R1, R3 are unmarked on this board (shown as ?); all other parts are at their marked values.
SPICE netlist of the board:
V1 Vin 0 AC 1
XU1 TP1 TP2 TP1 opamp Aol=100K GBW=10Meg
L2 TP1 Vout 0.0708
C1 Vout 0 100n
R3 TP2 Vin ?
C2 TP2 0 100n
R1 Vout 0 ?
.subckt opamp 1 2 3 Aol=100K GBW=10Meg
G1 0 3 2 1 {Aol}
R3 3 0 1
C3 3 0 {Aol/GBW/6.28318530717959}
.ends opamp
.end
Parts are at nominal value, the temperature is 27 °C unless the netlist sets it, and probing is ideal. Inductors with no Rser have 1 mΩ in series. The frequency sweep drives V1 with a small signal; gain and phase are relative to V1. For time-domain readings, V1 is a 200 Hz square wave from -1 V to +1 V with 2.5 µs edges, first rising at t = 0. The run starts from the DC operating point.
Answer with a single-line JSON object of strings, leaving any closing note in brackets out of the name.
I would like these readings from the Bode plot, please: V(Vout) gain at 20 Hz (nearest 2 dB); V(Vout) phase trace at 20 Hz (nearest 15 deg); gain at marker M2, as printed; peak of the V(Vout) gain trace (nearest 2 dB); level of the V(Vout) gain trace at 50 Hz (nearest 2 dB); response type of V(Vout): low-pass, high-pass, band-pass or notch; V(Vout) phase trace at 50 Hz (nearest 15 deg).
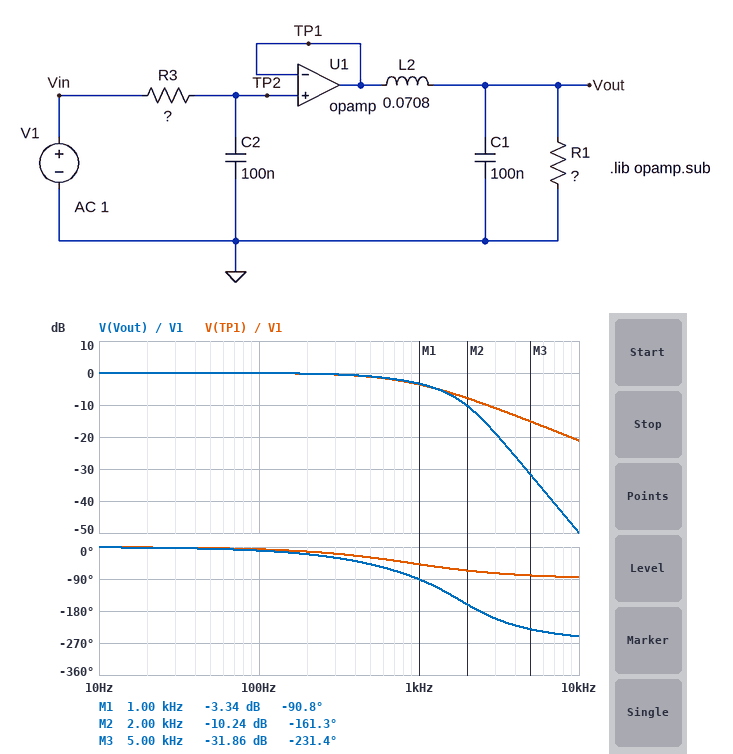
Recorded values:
{"V(Vout) gain at 20 Hz": "0 dB", "V(Vout) phase trace at 20 Hz": "0 deg", "gain at marker M2, as printed": "-10.24 dB", "peak of the V(Vout) gain trace": "0 dB", "level of the V(Vout) gain trace at 50 Hz": "0 dB", "response type of V(Vout): low-pass, high-pass, band-pass or notch": "low-pass", "V(Vout) phase trace at 50 Hz": "0 deg"}
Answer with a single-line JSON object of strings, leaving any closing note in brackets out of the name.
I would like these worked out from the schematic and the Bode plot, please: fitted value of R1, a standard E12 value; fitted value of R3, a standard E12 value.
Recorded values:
{"fitted value of R1, a standard E12 value": "680 Ω", "fitted value of R3, a standard E12 value": "1.8 kΩ"}
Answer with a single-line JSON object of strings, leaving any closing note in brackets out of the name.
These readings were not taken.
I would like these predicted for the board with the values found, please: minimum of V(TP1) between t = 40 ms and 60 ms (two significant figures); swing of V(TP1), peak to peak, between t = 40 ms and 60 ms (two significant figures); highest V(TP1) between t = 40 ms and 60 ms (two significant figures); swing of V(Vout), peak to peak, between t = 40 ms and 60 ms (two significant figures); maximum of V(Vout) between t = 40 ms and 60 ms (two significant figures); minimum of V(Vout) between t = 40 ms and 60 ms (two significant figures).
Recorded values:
{"minimum of V(TP1) between t = 40 ms and 60 ms": "-1.0 V", "swing of V(TP1), peak to peak, between t = 40 ms and 60 ms": "2.0 V", "highest V(TP1) between t = 40 ms and 60 ms": "1.0 V", "swing of V(Vout), peak to peak, between t = 40 ms and 60 ms": "2.0 V", "maximum of V(Vout) between t = 40 ms and 60 ms": "1.0 V", "minimum of V(Vout) between t = 40 ms and 60 ms": "-1.0 V"}
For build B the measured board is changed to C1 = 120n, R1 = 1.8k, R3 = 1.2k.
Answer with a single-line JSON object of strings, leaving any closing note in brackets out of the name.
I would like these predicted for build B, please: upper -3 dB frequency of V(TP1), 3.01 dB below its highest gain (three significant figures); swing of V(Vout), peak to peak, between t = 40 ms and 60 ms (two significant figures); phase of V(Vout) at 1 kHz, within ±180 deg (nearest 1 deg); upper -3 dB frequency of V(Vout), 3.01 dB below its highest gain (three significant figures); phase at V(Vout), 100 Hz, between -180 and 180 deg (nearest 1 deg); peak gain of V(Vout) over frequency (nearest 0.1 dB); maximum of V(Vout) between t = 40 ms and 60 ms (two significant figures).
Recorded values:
{"upper -3 dB frequency of V(TP1), 3.01 dB below its highest gain": "1.33 kHz", "swing of V(Vout), peak to peak, between t = 40 ms and 60 ms": "3.0 V", "phase of V(Vout) at 1 kHz, within ±180 deg": "-57 deg", "upper -3 dB frequency of V(Vout), 3.01 dB below its highest gain": "1.92 kHz", "phase at V(Vout), 100 Hz, between -180 and 180 deg": "-6 deg", "peak gain of V(Vout) over frequency": "3.6 dB", "maximum of V(Vout) between t = 40 ms and 60 ms": "1.5 V"}
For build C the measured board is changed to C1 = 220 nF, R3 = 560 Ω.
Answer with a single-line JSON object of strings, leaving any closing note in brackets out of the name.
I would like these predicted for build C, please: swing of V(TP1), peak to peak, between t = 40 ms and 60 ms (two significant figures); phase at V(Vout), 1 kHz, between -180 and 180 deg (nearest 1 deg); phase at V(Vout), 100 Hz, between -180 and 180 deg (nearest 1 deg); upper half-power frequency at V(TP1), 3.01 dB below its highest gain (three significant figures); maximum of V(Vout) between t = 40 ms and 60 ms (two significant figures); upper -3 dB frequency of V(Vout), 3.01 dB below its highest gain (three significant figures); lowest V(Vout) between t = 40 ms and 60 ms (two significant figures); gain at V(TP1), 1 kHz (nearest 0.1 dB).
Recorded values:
{"swing of V(TP1), peak to peak, between t = 40 ms and 60 ms": "2.0 V", "phase at V(Vout), 1 kHz, between -180 and 180 deg": "-79 deg", "phase at V(Vout), 100 Hz, between -180 and 180 deg": "-6 deg", "upper half-power frequency at V(TP1), 3.01 dB below its highest gain": "2.84 kHz", "maximum of V(Vout) between t = 40 ms and 60 ms": "1.4 V", "upper -3 dB frequency of V(Vout), 3.01 dB below its highest gain": "1.47 kHz", "lowest V(Vout) between t = 40 ms and 60 ms": "-1.4 V", "gain at V(TP1), 1 kHz": "-0.5 dB"}
